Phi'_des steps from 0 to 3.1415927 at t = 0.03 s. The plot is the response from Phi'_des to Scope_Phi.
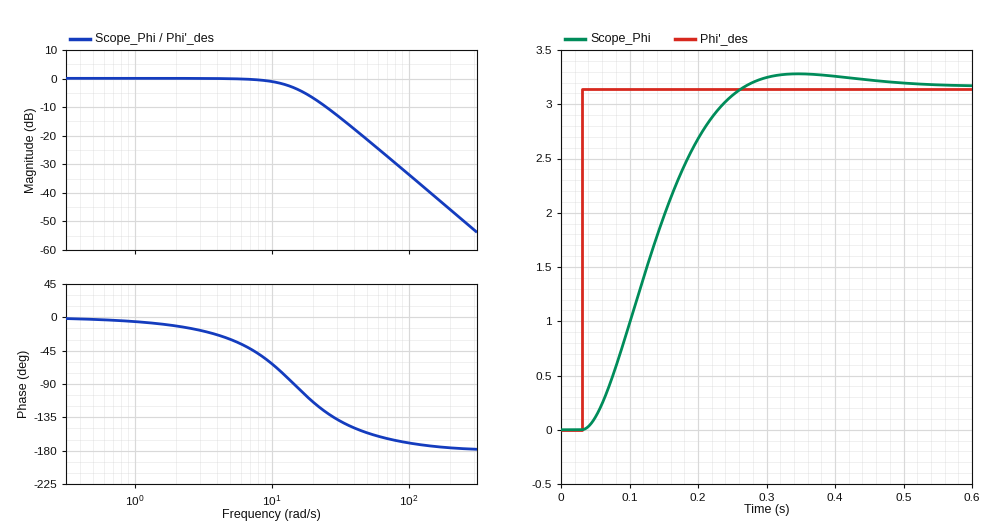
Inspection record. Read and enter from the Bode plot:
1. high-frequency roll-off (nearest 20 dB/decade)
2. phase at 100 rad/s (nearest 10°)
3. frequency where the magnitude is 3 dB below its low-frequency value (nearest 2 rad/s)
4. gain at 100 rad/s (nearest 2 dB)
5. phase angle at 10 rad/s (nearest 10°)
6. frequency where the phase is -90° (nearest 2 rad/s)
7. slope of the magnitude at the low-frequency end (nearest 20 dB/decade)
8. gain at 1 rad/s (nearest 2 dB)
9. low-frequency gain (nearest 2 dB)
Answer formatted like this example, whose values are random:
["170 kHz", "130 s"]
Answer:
["-40 dB/decade", "-170°", "14 rad/s", "-34 dB", "-60°", "14 rad/s", "0 dB/decade", "0 dB", "0 dB"]
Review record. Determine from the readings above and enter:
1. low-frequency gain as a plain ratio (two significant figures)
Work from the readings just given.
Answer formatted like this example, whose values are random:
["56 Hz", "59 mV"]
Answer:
["1.0"]
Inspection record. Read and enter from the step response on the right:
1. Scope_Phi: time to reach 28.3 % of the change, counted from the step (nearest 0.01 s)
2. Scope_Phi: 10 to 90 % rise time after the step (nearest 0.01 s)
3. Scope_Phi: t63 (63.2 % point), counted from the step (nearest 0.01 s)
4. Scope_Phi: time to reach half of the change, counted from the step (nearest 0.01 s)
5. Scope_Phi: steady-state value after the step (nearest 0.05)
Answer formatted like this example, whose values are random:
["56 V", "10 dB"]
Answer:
["0.07 s", "0.15 s", "0.12 s", "0.10 s", "3.15"]
